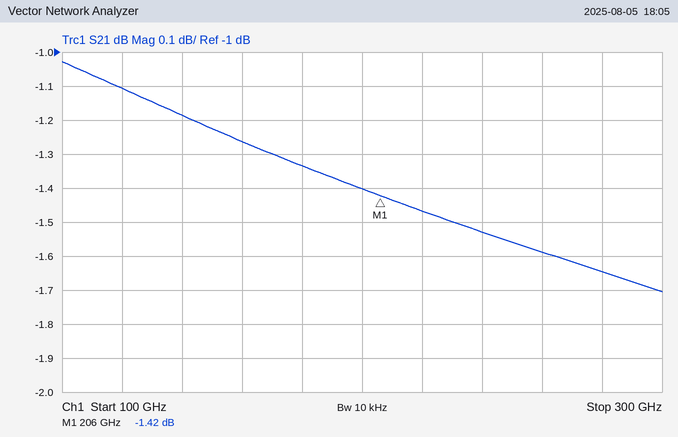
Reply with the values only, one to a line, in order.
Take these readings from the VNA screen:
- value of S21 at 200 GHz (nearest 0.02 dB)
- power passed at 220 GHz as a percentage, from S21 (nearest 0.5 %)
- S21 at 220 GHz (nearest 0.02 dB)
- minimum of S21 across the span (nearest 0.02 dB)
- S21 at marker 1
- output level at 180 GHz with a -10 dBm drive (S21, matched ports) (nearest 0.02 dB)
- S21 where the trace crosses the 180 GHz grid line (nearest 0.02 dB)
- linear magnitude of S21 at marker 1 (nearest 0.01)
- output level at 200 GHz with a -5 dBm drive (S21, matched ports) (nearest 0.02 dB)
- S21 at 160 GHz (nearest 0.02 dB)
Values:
-1.40 dB
71.5 %
-1.46 dB
-1.70 dB
-1.42 dB
-11.34 dBm
-1.34 dB
0.85
-6.40 dBm
-1.26 dB
